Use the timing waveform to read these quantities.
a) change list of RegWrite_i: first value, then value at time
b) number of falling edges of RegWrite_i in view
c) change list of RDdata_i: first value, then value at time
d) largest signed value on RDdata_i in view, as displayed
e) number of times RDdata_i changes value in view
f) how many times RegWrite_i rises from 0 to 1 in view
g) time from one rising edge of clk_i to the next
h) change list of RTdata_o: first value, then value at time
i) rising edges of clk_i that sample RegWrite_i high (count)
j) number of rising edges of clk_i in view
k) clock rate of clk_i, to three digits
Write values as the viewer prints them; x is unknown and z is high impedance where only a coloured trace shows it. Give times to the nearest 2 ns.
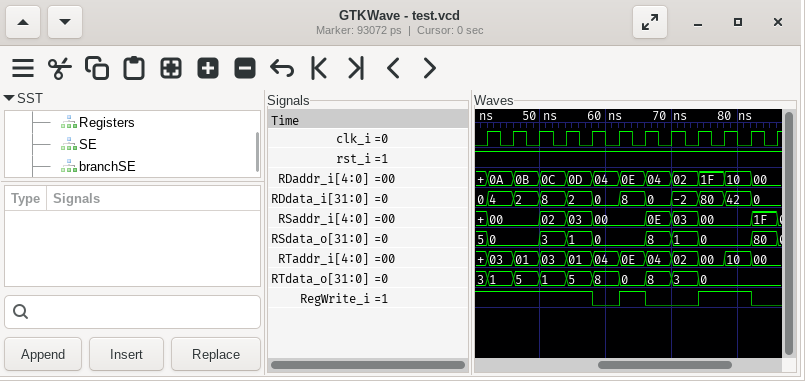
1, 0 at 58 ns, 1 at 62 ns, 0 at 66 ns, 1 at 74 ns, 0 at 82 ns
3
0, 4 at 42 ns, 2 at 46 ns, 8 at 50 ns, 2 at 54 ns, 0 at 58 ns, 8 at 62 ns, 0 at 66 ns, -2 at 70 ns, 80 at 74 ns, 42 at 78 ns, 0 at 82 ns
80
11
2
4 ns
3, 1 at 42 ns, 5 at 46 ns, 1 at 50 ns, 5 at 54 ns, 8 at 58 ns, 0 at 62 ns, 8 at 66 ns, 3 at 70 ns, 0 at 74 ns
8
12
250 MHz
